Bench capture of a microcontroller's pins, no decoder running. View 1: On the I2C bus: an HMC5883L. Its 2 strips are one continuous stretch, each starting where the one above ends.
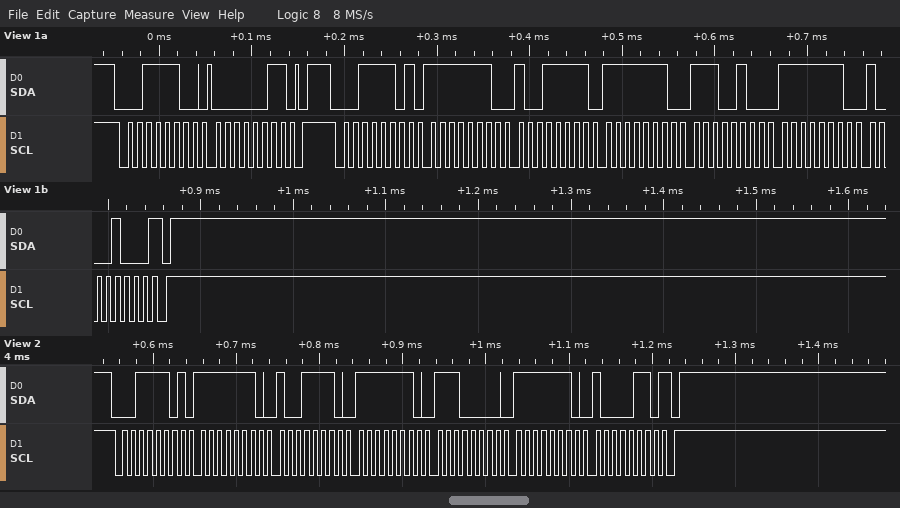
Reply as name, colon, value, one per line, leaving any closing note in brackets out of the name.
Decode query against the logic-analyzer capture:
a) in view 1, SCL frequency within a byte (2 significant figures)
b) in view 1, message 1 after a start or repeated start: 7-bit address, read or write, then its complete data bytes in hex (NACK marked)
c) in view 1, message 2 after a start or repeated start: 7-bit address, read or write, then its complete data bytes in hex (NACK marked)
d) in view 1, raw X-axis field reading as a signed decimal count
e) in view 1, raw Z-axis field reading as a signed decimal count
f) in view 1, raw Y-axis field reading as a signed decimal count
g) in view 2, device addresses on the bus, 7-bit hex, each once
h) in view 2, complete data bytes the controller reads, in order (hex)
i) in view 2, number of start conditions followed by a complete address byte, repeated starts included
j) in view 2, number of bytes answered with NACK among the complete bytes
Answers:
in view 1, SCL frequency within a byte: 100 kHz
in view 1, message 1 after a start or repeated start: 7-bit address, read or write, then its complete data bytes in hex: 0x1E write: 03
in view 1, message 2 after a start or repeated start: 7-bit address, read or write, then its complete data bytes in hex: 0x1E read: FE 9F FE E4 FE 88 NACK
in view 1, raw X-axis field reading as a signed decimal count: -353
in view 1, raw Z-axis field reading as a signed decimal count: -284
in view 1, raw Y-axis field reading as a signed decimal count: -376
in view 2, device addresses on the bus, 7-bit hex, each once: 0x1E
in view 2, complete data bytes the controller reads, in order: FE 9E FE E0 FE 86
in view 2, number of start conditions followed by a complete address byte, repeated starts included: 1
in view 2, number of bytes answered with NACK among the complete bytes: 1
